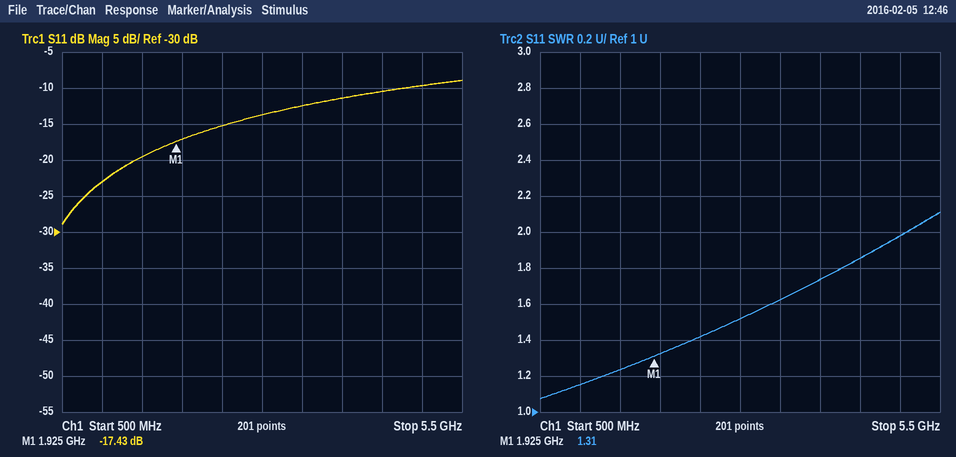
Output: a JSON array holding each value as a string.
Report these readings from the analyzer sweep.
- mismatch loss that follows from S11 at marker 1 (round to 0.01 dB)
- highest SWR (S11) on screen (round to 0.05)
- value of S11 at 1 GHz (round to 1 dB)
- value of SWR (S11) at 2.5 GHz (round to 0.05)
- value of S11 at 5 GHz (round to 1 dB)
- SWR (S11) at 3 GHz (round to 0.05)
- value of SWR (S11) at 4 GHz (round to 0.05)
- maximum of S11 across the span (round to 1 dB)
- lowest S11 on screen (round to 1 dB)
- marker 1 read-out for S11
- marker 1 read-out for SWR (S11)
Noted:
["0.08 dB", "2.10", "-23 dB", "1.40", "-10 dB", "1.50", "1.75", "-9 dB", "-29 dB", "-17.43 dB", "1.31"]
